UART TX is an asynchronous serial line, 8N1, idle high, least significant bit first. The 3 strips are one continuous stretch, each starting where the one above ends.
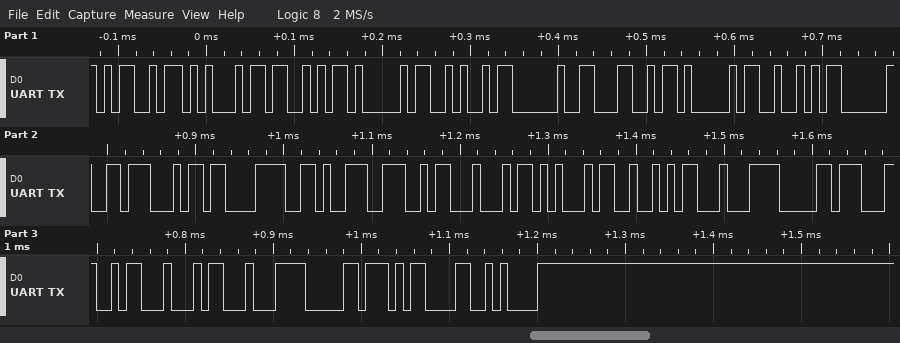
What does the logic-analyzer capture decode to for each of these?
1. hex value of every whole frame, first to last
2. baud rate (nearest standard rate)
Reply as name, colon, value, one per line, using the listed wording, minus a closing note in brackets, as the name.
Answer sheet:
hex value of every whole frame, first to last: 4D 45 53 41 4A 20 4C 41 52 20 47 C3 96 4E 44 45 52 C4 B0 4C 44 C4 B0 0D 0A
baud rate: 115200 baud
